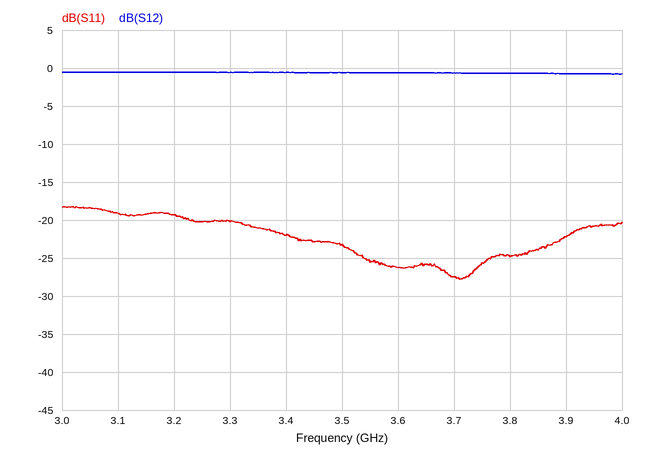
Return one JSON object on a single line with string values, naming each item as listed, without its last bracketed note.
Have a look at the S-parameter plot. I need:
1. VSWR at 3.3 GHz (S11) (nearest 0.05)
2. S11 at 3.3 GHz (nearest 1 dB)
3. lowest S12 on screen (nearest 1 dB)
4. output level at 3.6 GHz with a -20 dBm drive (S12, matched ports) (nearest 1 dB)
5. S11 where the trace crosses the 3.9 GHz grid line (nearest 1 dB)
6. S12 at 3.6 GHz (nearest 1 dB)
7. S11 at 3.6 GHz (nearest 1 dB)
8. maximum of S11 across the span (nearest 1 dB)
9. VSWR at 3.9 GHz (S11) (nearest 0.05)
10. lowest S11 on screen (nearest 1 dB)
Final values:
{"VSWR at 3.3 GHz (S11)": "1.20", "S11 at 3.3 GHz": "-20 dB", "lowest S12 on screen": "-1 dB", "output level at 3.6 GHz with a -20 dBm drive (S12, matched ports)": "-21 dBm", "S11 where the trace crosses the 3.9 GHz grid line": "-22 dB", "S12 at 3.6 GHz": "-1 dB", "S11 at 3.6 GHz": "-26 dB", "maximum of S11 across the span": "-18 dB", "VSWR at 3.9 GHz (S11)": "1.15", "lowest S11 on screen": "-28 dB"}
